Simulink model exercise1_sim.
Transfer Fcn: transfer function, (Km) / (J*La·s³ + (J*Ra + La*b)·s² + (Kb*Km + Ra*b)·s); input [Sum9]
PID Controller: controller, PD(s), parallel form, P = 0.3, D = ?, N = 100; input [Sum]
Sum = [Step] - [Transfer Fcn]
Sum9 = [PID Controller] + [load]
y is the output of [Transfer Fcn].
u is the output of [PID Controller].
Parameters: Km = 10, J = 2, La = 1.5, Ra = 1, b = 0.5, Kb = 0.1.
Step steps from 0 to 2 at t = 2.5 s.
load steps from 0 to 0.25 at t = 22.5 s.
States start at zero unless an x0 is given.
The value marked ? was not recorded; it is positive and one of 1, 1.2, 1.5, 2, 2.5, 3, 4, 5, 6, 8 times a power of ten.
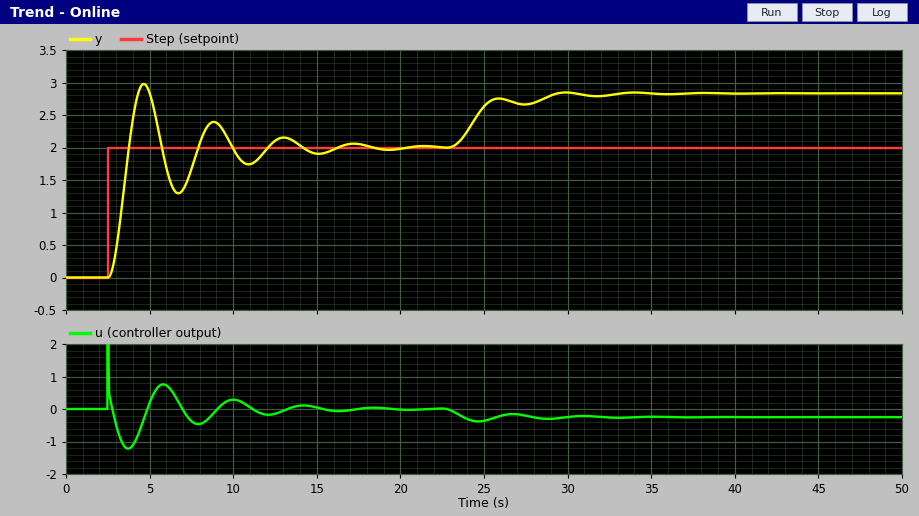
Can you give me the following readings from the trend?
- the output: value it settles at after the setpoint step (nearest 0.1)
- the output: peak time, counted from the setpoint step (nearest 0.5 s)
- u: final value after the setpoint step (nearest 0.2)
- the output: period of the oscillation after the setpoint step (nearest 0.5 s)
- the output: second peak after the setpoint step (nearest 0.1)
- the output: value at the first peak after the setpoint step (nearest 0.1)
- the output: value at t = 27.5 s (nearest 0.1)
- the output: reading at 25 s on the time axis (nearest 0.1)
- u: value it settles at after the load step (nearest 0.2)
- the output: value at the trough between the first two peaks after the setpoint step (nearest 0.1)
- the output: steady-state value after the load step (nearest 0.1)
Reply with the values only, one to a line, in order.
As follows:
2.0
2.0 s
0.0
4.0 s
2.4
3.0
2.7
2.6
-0.2
1.3
2.8
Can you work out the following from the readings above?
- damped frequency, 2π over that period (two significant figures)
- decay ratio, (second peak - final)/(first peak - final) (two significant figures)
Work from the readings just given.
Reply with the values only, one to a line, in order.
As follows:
1.6 rad/s
0.40
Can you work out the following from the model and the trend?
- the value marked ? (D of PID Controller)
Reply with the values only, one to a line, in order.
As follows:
0.6
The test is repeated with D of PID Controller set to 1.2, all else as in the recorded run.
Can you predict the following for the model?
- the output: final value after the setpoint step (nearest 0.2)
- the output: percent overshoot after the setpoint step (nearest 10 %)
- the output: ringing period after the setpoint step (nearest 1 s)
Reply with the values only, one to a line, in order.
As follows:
2.0
50 %
3 s
